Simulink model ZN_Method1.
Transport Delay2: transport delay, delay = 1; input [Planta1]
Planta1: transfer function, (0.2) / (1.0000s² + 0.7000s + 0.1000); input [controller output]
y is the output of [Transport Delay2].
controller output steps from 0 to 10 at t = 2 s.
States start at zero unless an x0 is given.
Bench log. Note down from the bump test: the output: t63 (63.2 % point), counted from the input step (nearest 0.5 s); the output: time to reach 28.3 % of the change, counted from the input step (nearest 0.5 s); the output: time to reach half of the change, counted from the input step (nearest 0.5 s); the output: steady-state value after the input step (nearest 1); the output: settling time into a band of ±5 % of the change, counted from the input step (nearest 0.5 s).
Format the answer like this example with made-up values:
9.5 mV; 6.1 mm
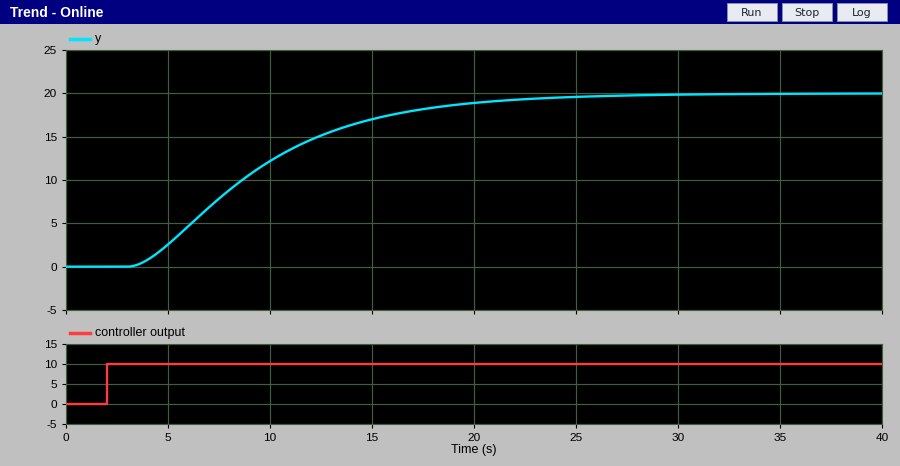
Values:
8.5 s; 4.5 s; 6.5 s; 20; 18.5 s
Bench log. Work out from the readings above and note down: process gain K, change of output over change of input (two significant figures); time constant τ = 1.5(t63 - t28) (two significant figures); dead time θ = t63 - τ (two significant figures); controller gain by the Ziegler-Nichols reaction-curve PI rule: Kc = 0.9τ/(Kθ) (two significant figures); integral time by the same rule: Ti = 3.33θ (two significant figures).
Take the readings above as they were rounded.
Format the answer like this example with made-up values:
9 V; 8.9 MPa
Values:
2.0; 6.0 s; 2.5 s; 1.1; 8.3 s
